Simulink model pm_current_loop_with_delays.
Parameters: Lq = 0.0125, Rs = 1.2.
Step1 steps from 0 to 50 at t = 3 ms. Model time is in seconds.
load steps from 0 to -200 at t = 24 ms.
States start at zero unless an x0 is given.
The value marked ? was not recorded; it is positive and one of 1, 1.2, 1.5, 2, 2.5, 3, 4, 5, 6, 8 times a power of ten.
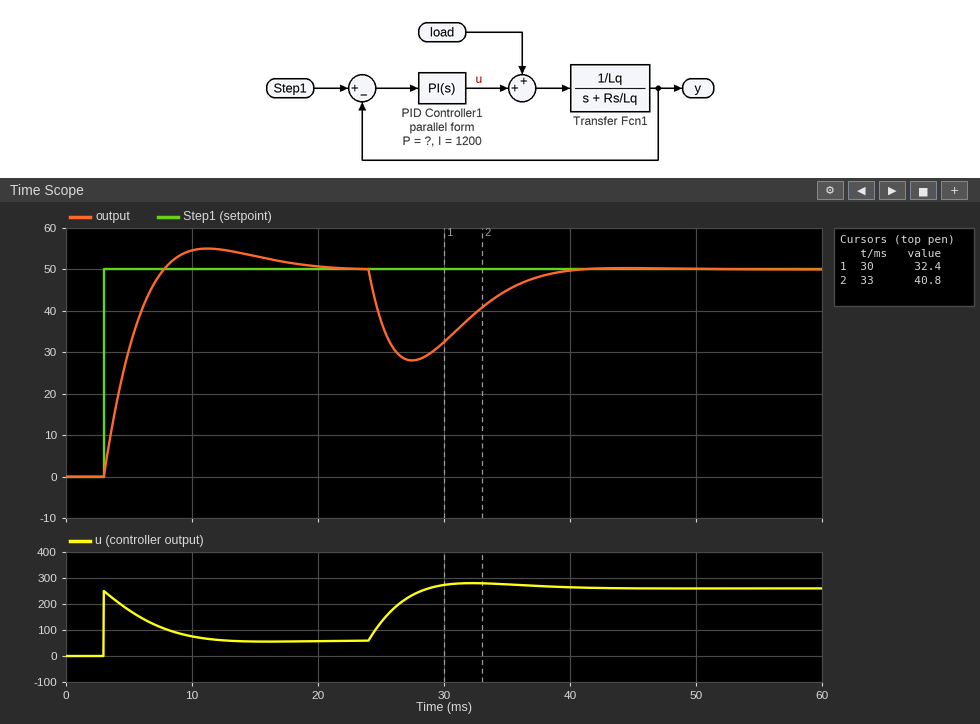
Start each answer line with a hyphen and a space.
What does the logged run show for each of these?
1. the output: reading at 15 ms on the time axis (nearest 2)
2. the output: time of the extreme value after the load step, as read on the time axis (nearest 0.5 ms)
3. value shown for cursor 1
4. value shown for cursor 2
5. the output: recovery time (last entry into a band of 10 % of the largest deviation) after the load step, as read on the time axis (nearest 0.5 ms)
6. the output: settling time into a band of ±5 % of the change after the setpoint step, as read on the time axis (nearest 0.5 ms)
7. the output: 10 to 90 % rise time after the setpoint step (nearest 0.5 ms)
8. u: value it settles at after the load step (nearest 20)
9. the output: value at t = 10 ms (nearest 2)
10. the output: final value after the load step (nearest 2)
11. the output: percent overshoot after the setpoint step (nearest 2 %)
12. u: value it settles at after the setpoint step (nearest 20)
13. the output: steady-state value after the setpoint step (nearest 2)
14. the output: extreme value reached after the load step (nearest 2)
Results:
- 54
- 27.5 ms
- 32.4
- 40.8
- 37.0 ms
- 16.0 ms
- 3.5 ms
- 260
- 54
- 50
- 10 %
- 60
- 50
- 28
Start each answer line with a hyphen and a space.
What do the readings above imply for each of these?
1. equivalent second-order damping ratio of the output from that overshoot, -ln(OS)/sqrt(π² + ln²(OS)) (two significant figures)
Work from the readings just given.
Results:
- 0.59
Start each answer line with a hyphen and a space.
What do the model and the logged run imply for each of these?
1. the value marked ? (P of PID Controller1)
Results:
- 5
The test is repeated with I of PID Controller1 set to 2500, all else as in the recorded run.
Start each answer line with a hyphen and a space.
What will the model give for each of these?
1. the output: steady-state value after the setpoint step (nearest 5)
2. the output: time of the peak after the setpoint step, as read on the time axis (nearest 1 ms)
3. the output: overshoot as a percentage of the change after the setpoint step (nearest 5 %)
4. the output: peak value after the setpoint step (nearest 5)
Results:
- 50
- 9 ms
- 20 %
- 60
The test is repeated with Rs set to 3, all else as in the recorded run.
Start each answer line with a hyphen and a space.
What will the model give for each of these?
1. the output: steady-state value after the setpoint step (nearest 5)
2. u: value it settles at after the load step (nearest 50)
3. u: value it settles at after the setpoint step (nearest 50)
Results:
- 50
- 350
- 150
